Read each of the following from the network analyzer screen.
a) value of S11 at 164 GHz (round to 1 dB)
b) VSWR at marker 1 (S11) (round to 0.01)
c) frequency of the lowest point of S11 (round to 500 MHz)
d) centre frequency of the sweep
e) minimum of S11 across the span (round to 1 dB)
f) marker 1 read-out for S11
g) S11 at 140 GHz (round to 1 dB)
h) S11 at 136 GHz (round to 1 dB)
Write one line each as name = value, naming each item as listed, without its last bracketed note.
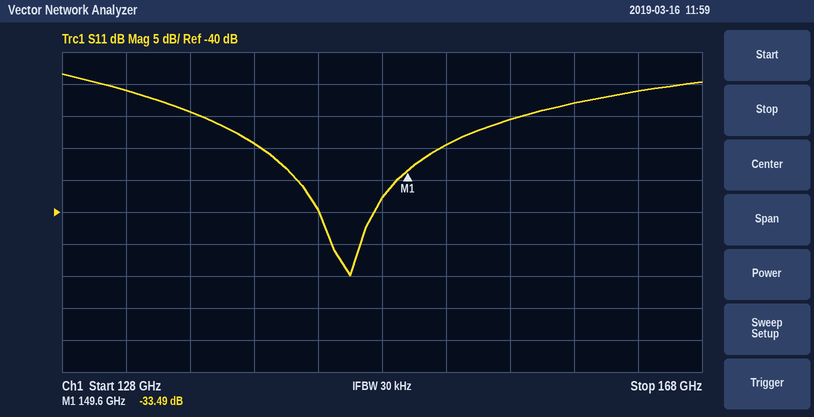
value of S11 at 164 GHz = -21 dB
VSWR at marker 1 (S11) = 1.04
frequency of the lowest point of S11 = 146.0 GHz
centre frequency of the sweep = 148 GHz
minimum of S11 across the span = -50 dB
marker 1 read-out for S11 = -33.49 dB
S11 at 140 GHz = -29 dB
S11 at 136 GHz = -24 dB
